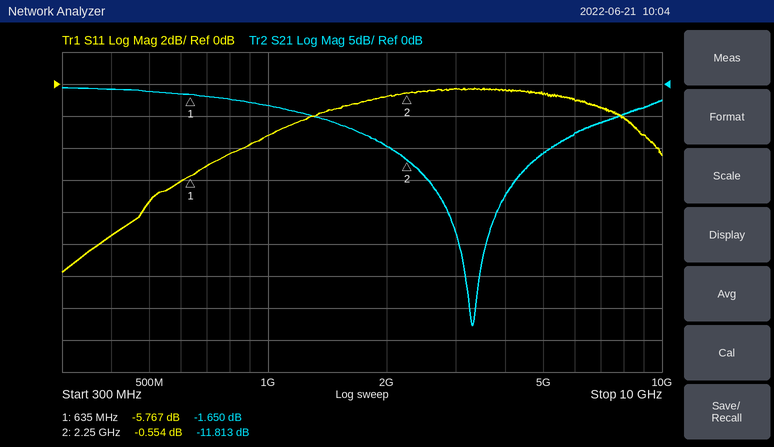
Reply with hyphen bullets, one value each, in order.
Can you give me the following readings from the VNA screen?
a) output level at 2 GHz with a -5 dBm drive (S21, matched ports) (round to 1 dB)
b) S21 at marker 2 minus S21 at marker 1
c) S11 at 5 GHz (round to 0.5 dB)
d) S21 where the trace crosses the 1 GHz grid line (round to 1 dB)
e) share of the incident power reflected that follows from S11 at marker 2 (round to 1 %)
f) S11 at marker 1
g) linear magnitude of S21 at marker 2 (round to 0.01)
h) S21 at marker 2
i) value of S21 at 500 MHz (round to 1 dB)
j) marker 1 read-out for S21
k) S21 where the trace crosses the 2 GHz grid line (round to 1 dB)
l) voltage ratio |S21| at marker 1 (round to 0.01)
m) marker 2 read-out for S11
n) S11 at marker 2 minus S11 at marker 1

- -15 dBm
- -10.163 dB
- -0.5 dB
- -3 dB
- 88 %
- -5.767 dB
- 0.26
- -11.813 dB
- -1 dB
- -1.650 dB
- -10 dB
- 0.83
- -0.554 dB
- 5.213 dB
